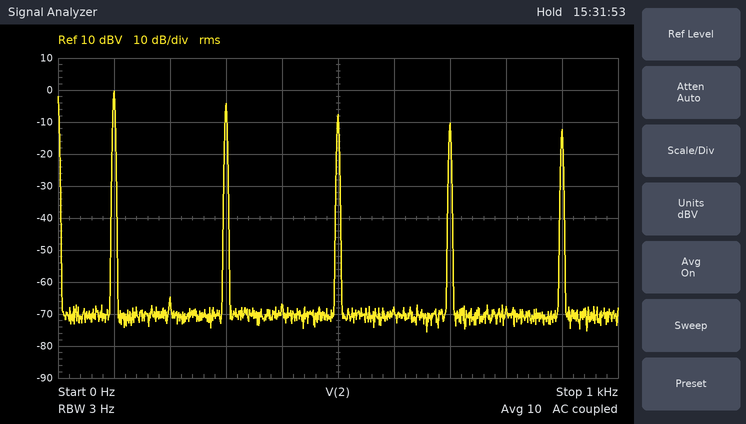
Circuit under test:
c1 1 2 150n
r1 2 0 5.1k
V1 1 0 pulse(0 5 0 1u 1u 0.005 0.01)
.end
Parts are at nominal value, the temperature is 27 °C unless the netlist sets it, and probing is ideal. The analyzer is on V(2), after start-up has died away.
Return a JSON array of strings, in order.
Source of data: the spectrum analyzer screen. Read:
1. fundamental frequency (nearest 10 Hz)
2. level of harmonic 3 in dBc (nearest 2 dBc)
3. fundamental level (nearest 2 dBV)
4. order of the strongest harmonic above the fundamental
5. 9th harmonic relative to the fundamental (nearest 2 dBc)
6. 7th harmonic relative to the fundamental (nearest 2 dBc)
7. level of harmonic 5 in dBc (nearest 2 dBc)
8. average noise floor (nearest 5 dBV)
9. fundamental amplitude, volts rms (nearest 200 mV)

["100 Hz", "-4 dBc", "0 dBV", "3", "-12 dBc", "-10 dBc", "-8 dBc", "-70 dBV", "1.0 V"]
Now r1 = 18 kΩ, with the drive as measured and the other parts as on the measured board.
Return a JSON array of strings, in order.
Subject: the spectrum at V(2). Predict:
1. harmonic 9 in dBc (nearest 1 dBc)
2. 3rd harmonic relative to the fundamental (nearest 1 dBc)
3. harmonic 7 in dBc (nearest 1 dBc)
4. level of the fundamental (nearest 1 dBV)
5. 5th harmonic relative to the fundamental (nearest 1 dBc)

["-18 dBc", "-8 dBc", "-16 dBc", "6 dBV", "-13 dBc"]
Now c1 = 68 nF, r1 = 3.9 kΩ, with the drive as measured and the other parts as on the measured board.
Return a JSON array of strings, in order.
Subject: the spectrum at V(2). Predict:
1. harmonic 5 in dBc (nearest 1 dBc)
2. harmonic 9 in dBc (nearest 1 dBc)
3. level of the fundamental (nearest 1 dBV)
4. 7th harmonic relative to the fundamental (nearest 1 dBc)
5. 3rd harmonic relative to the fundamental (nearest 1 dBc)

["-2 dBc", "-5 dBc", "-9 dBV", "-4 dBc", "-1 dBc"]
